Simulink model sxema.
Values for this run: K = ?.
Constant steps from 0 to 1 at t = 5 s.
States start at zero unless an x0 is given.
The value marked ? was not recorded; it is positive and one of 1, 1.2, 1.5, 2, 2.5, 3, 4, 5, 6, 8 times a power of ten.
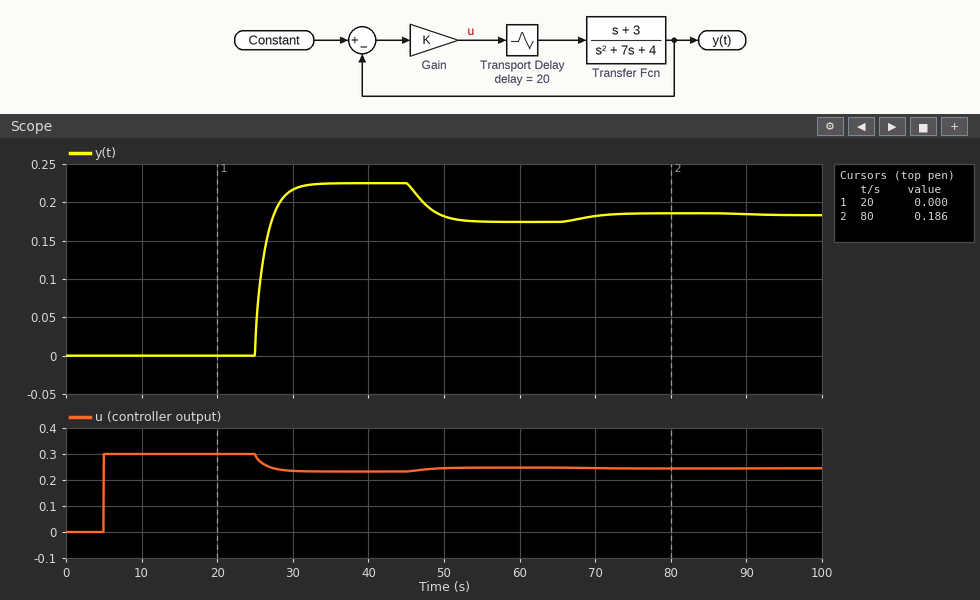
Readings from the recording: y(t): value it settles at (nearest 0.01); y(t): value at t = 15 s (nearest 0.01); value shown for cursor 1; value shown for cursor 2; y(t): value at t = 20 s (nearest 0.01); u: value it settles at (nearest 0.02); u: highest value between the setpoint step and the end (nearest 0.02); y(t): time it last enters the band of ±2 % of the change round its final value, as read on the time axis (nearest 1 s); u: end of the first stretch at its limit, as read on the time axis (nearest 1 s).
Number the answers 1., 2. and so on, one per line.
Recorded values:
1. 0.18
2. 0.00
3. 0.000
4. 0.186
5. 0.00
6. 0.24
7. 0.30
8. 69 s
9. 25 s
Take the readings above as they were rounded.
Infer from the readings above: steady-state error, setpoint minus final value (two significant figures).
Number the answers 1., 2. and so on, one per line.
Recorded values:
1. 0.82
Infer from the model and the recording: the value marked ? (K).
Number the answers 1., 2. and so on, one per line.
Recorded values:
1. 0.3
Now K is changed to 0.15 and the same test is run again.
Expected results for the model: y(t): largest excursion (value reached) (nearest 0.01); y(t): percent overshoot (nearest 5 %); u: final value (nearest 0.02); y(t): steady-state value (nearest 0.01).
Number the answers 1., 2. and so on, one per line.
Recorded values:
1. 0.11
2. 10 %
3. 0.14
4. 0.10
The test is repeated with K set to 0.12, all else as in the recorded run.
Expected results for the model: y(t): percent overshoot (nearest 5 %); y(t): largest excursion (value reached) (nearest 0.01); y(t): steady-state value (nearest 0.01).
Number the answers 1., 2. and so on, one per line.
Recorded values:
1. 10 %
2. 0.09
3. 0.08
